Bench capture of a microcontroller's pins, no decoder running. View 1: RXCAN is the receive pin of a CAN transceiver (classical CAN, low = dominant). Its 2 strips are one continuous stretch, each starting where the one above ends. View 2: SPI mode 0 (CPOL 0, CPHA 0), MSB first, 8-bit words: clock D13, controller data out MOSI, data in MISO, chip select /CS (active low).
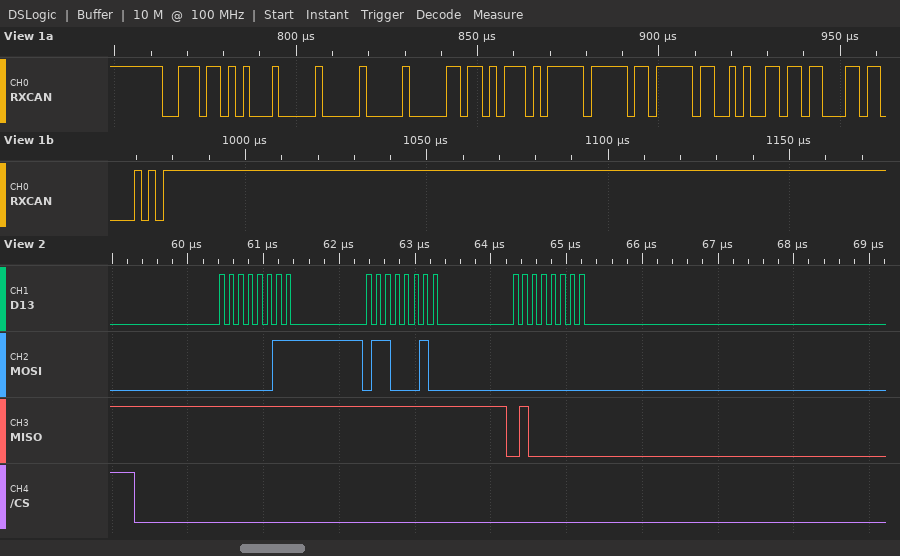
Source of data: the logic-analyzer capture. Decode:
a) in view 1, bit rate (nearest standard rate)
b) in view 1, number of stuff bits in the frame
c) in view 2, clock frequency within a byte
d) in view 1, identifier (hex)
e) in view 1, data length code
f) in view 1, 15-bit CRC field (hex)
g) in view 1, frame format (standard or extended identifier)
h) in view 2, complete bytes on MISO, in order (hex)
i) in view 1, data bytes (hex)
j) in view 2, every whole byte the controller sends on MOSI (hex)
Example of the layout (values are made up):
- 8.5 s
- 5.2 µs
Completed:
- 500 kbit/s
- 7
- 8 MHz
- 0x3B5
- 8
- 0x46C2
- standard
- FF FF 40
- 00 00 5A EB FF DF CA 6D
- 03 62 00
